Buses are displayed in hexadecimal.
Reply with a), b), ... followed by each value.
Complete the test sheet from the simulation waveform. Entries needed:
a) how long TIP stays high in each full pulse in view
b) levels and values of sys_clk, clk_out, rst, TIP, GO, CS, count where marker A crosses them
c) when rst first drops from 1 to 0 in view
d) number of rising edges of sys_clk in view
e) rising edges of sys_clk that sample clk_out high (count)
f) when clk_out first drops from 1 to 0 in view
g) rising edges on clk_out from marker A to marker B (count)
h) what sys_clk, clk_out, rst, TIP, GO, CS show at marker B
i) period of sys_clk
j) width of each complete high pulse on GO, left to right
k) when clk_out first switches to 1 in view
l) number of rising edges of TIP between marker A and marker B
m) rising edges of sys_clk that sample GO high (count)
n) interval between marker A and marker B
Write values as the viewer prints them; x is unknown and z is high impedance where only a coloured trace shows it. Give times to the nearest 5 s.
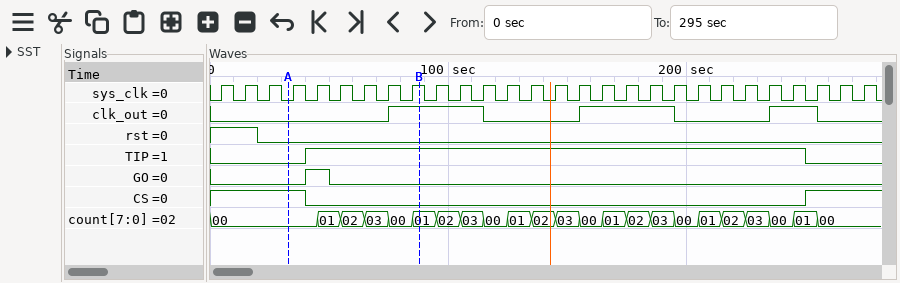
a) 210 s
b) sys_clk=0, clk_out=0, rst=0, TIP=0, GO=0, CS=1, count=00
c) 20 s
d) 28
e) 10
f) 115 s
g) 1
h) sys_clk=1, clk_out=1, rst=0, TIP=1, GO=0, CS=0
i) 10 s
j) 10 s
k) 75 s
l) 1
m) 1
n) 55 s
